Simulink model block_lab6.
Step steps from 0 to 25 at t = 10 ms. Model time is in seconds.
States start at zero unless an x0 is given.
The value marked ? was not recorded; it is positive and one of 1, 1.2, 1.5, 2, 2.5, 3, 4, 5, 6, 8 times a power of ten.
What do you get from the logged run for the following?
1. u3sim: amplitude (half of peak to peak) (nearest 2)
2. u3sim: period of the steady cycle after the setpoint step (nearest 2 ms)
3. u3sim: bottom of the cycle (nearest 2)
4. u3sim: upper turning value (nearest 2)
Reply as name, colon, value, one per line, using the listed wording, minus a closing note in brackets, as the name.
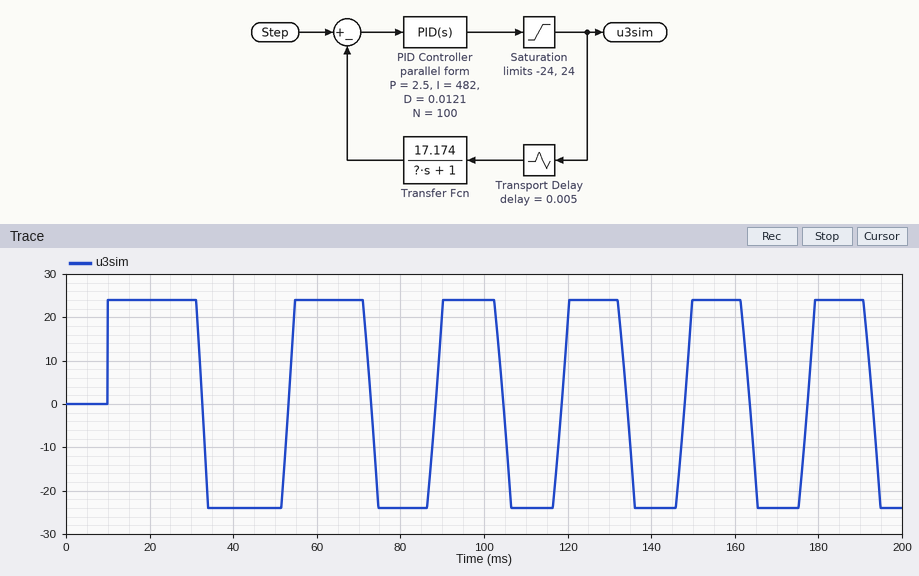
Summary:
u3sim: amplitude (half of peak to peak): 24
u3sim: period of the steady cycle after the setpoint step: 30 ms
u3sim: bottom of the cycle: -24
u3sim: upper turning value: 24
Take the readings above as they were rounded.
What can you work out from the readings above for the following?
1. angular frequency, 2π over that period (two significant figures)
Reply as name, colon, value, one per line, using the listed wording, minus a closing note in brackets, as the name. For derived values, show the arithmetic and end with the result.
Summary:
angular frequency, 2π over that period: 2π / 30 = 0.21 rad/ms
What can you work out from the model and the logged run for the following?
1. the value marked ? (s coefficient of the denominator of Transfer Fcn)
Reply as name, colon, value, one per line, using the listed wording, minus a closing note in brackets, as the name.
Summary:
the value marked ?: 0.15
